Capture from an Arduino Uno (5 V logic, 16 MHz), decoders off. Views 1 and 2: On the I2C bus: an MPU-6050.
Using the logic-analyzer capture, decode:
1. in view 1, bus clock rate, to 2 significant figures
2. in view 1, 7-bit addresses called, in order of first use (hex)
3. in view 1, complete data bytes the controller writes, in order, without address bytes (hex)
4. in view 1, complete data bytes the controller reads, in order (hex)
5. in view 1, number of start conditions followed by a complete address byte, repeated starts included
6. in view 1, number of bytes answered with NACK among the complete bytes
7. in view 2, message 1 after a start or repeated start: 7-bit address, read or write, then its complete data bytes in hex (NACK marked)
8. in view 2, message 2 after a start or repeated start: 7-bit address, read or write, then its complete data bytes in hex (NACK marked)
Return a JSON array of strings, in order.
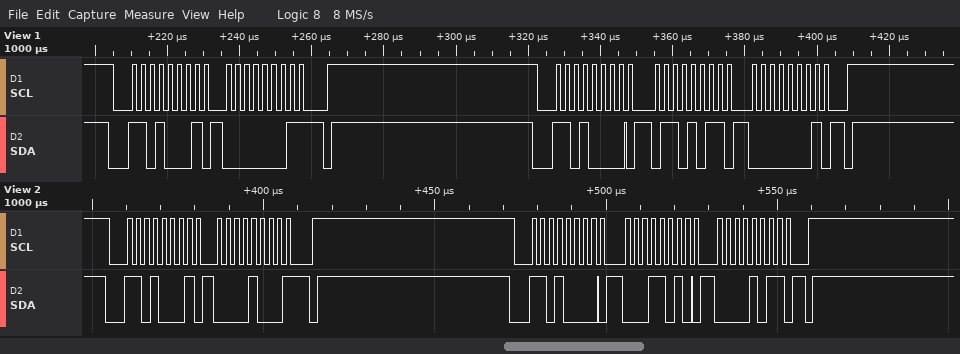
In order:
["400 kHz", "0x68", "6B 01", "01", "2", "1", "0x68 read: 08 NACK", "0x68 write: 1A 0B"]
